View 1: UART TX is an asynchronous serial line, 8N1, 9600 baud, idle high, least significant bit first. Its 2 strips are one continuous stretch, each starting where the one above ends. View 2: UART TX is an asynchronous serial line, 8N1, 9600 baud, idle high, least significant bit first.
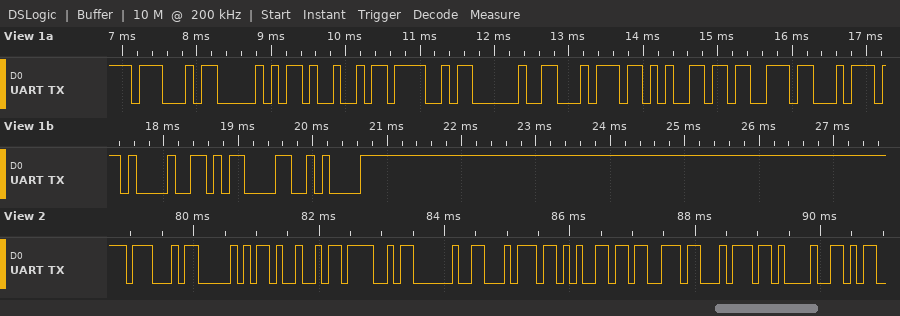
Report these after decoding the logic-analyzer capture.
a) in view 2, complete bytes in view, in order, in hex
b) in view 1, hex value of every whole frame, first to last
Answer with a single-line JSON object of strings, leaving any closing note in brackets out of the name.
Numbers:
{"in view 2, complete bytes in view, in order, in hex": "47 50 49 4F 20 74 65 73 74 21", "in view 1, hex value of every whole frame, first to last": "0x47 0x50 0x49 0x4F 0x20 0x74 0x65 0x73 0x74 0x21 0x0D 0x0A"}
